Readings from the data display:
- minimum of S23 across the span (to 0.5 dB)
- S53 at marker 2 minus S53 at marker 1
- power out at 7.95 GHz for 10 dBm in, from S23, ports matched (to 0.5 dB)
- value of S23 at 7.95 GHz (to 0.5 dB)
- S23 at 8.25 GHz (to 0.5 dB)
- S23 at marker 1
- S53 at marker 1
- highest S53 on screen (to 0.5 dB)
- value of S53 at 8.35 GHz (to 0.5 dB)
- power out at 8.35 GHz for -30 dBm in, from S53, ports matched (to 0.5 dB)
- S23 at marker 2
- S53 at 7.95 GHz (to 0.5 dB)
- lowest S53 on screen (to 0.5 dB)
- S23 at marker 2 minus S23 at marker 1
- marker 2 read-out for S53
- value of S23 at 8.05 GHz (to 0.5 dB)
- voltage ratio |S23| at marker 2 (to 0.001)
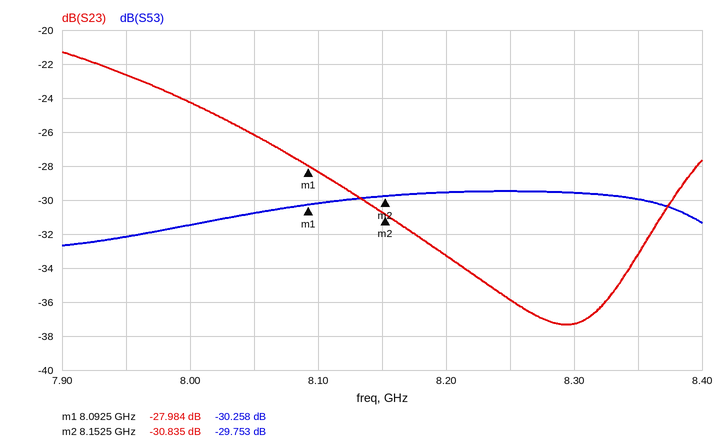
-37.5 dB
0.505 dB
-12.5 dBm
-22.5 dB
-36.0 dB
-27.984 dB
-30.258 dB
-29.5 dB
-30.0 dB
-60.0 dBm
-30.835 dB
-32.0 dB
-32.5 dB
-2.851 dB
-29.753 dB
-26.0 dB
0.029
